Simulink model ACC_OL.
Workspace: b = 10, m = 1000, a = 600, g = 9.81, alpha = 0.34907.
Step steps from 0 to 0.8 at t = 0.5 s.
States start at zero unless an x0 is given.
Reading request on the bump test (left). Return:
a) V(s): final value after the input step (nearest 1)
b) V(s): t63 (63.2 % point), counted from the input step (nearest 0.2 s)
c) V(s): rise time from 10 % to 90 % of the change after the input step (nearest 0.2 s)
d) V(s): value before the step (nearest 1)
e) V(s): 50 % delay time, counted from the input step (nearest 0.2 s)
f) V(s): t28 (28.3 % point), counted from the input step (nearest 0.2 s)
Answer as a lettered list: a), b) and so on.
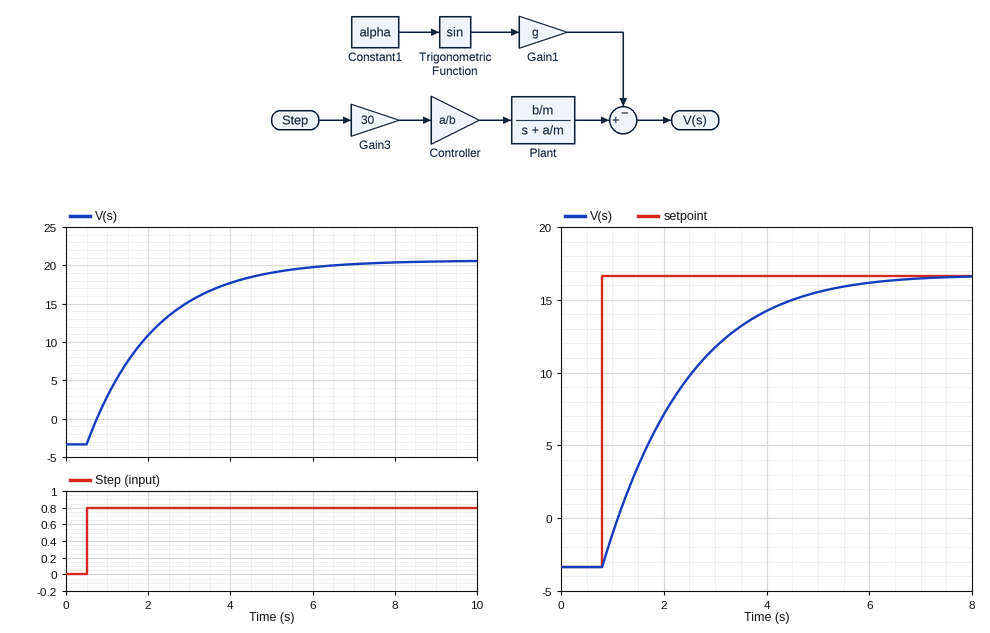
a) 21
b) 1.6 s
c) 3.6 s
d) -3
e) 1.2 s
f) 0.6 s
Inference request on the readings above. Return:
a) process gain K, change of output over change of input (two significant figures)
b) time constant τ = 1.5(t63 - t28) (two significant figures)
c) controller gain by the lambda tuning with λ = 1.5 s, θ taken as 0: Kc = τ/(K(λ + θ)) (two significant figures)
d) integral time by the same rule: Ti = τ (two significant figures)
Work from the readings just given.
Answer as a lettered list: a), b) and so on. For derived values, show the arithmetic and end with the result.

a) (21 - (-3)) / 0.8 = 30
b) 1.5 × (1.6 - 0.6) = 1.5 s
c) 1.5 / (30 × (1.5 + 0)) = 0.033
d) 1.5 s
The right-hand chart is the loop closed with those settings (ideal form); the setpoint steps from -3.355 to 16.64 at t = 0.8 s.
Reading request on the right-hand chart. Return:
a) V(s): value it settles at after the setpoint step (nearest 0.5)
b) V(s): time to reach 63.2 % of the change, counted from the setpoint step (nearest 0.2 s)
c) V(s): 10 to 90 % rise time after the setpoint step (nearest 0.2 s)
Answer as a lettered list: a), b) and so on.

a) 16.5
b) 1.6 s
c) 3.2 s
